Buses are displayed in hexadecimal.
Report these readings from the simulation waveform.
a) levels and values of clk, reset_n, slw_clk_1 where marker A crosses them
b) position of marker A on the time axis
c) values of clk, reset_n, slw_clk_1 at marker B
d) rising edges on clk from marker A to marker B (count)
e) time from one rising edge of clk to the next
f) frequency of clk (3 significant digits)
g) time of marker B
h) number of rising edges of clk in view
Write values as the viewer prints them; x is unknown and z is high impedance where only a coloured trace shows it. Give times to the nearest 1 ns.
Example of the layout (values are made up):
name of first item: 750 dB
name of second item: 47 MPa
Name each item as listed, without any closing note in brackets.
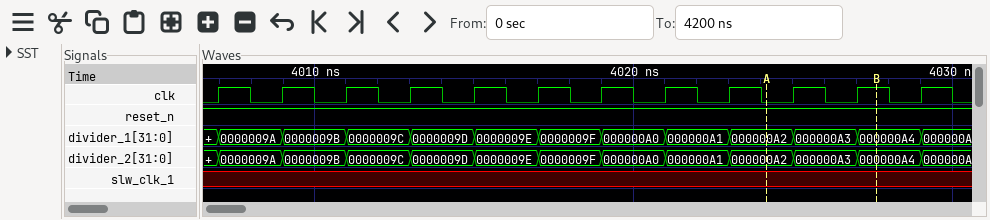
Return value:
levels and values of clk, reset_n, slw_clk_1 where marker A crosses them: clk=0, reset_n=1, slw_clk_1=x
position of marker A on the time axis: 4024 ns
values of clk, reset_n, slw_clk_1 at marker B: clk=1, reset_n=1, slw_clk_1=x
rising edges on clk from marker A to marker B: 2
time from one rising edge of clk to the next: 2 ns
frequency of clk: 500 MHz
time of marker B: 4028 ns
number of rising edges of clk in view: 12
